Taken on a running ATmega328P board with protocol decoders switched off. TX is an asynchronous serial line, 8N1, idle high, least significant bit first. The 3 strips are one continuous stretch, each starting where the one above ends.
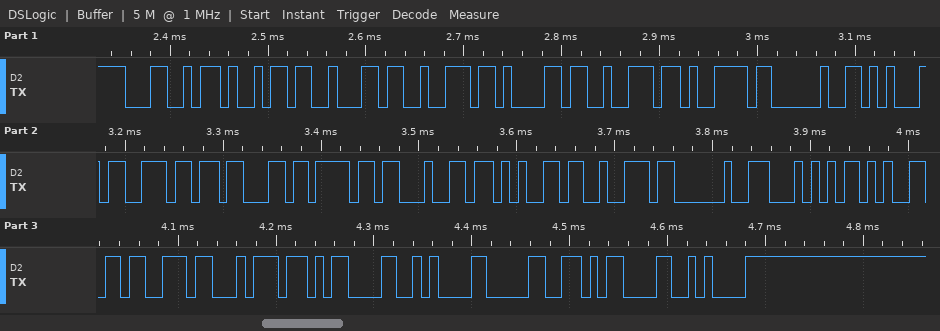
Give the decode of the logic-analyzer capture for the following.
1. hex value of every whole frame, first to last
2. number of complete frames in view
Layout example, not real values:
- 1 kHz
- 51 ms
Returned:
- 4C 69 62 72 61 72 79 20 45 6E 63 6F 64 65 72 20 54 65 73 74 0D 0A 30 0D 0A
- 25
